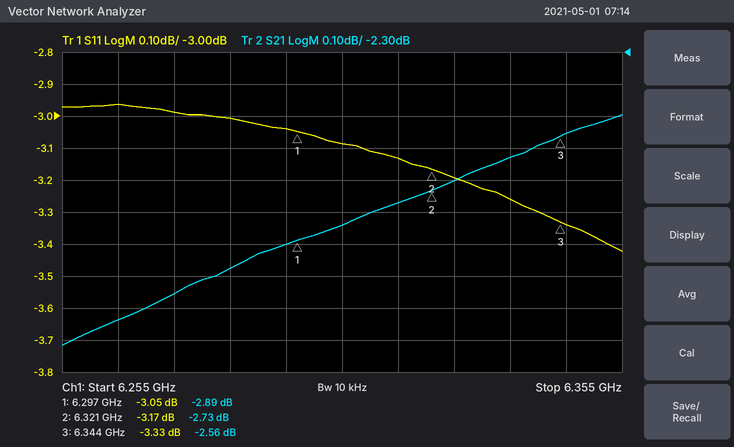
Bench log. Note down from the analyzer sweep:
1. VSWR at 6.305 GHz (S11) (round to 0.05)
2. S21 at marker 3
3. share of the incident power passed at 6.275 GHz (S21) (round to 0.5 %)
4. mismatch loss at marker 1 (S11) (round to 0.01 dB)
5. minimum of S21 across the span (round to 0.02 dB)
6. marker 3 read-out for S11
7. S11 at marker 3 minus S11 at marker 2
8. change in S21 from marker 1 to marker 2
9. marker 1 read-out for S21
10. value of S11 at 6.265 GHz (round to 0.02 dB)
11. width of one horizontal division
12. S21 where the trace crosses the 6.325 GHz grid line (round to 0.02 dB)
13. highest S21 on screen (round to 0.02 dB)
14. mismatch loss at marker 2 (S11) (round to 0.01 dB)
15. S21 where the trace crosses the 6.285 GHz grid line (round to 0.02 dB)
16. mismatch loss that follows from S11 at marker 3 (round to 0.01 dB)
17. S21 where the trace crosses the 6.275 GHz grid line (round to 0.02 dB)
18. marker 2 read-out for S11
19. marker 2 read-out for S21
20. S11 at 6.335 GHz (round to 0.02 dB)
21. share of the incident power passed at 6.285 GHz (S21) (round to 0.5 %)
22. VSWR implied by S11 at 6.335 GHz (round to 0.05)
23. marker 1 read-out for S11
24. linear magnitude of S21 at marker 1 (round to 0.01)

5.70
-2.56 dB
49.5 %
2.97 dB
-3.22 dB
-3.33 dB
-0.16 dB
0.16 dB
-2.89 dB
-2.96 dB
10 MHz
-2.70 dB
-2.50 dB
2.86 dB
-2.98 dB
2.71 dB
-3.06 dB
-3.17 dB
-2.73 dB
-3.26 dB
50.5 %
5.40
-3.05 dB
0.72
